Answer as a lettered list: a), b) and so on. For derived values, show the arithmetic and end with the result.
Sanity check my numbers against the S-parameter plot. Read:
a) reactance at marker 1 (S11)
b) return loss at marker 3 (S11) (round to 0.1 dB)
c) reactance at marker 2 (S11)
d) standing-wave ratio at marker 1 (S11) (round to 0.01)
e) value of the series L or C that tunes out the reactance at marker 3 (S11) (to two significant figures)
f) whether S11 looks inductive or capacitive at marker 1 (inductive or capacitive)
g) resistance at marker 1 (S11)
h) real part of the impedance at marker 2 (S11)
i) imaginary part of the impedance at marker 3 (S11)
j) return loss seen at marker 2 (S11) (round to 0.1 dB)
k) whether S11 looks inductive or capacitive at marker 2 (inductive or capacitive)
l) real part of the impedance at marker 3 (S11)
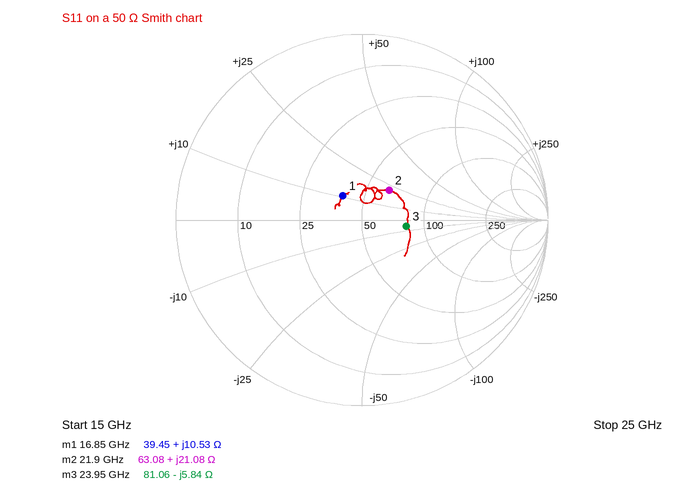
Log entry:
a) +10.53 Ω
b) 12.4 dB
c) +21.08 Ω
d) 1.40
e) L = 5.84 Ω/(2π × 23.95 GHz) ≈ 39 pH
f) inductive
g) 39.45 Ω
h) 63.08 Ω
i) -5.84 Ω
j) 13.3 dB
k) inductive
l) 81.06 Ω
